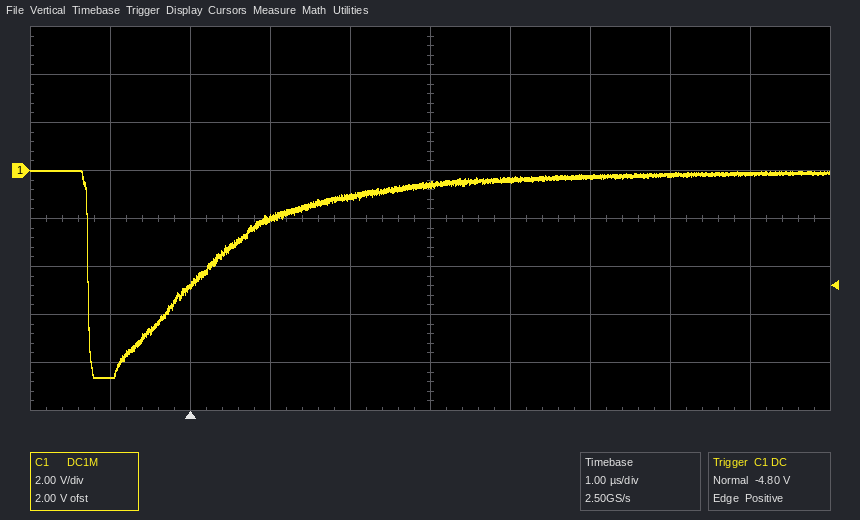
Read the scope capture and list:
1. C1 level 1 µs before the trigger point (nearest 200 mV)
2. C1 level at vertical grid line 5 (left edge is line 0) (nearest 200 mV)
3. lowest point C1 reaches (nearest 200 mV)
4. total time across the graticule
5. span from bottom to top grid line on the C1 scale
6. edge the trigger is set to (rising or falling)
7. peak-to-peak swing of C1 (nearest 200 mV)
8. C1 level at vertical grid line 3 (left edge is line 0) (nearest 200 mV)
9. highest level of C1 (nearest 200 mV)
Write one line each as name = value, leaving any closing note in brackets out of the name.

C1 level 1 µs before the trigger point = -8.6 V
C1 level at vertical grid line 5 (left edge is line 0) = -600 mV
lowest point C1 reaches = -8.6 V
total time across the graticule = 10 µs
span from bottom to top grid line on the C1 scale = 16 V
edge the trigger is set to = rising
peak-to-peak swing of C1 = 8.6 V
C1 level at vertical grid line 3 (left edge is line 0) = -2.0 V
highest level of C1 = 0.0 V
